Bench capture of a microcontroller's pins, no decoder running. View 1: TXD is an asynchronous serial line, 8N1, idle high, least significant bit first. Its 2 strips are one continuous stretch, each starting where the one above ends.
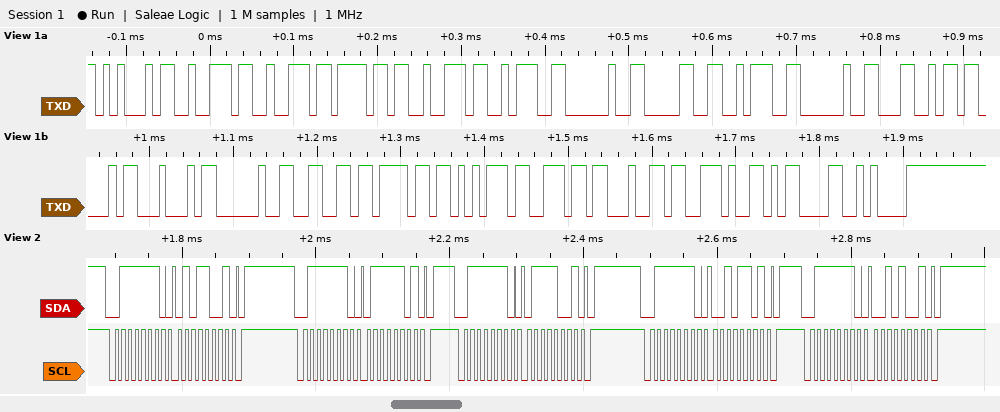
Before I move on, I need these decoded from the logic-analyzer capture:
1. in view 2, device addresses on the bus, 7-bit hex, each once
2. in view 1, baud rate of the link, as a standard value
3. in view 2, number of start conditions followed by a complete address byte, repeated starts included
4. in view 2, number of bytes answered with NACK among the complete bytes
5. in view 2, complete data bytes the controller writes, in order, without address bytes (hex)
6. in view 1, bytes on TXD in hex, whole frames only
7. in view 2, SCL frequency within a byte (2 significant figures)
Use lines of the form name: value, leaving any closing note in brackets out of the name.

in view 2, device addresses on the bus, 7-bit hex, each once: 0x3F
in view 1, baud rate of the link, as a standard value: 115200 baud
in view 2, number of start conditions followed by a complete address byte, repeated starts included: 5
in view 2, number of bytes answered with NACK among the complete bytes: 0
in view 2, complete data bytes the controller writes, in order, without address bytes: 59 7D 79 2D 29
in view 1, bytes on TXD in hex, whole frames only: 0x45 0x72 0x72 0x6F 0x72 0x3A 0x20 0x30 0x3A 0x20 0x4C 0x43 0x44 0x20 0x66 0x6F 0x75 0x6E 0x64 0x2E 0x0D 0x0A
in view 2, SCL frequency within a byte: 100 kHz
